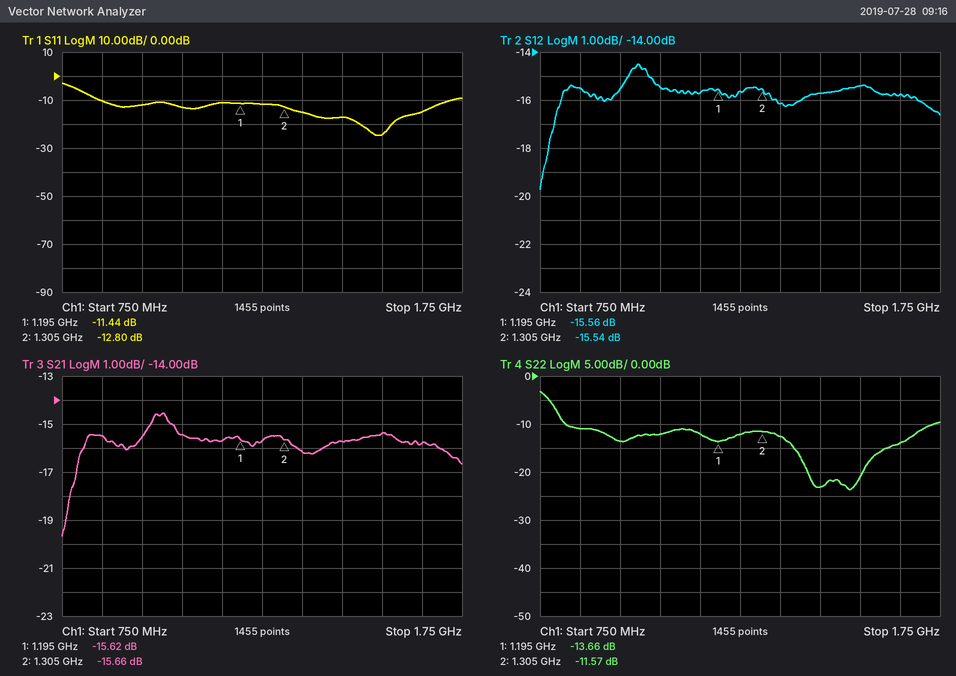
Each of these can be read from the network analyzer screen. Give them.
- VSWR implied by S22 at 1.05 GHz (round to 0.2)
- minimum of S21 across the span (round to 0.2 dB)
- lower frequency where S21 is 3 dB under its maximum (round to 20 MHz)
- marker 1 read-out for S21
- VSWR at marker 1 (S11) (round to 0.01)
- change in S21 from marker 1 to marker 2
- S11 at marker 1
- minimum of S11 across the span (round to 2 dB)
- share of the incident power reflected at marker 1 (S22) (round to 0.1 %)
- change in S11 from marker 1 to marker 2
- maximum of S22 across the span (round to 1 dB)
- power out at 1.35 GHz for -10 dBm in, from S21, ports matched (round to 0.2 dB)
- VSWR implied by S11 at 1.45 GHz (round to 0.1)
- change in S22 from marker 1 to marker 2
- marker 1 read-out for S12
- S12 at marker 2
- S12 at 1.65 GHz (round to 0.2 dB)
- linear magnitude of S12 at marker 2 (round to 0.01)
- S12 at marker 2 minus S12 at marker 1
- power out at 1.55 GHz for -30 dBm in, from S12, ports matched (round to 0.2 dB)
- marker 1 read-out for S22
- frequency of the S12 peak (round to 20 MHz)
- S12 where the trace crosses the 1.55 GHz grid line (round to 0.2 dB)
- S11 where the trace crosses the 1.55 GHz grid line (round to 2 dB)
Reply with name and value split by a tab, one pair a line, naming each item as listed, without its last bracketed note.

VSWR implied by S22 at 1.05 GHz	1.6
minimum of S21 across the span	-19.6 dB
lower frequency where S21 is 3 dB under its maximum	780 MHz
marker 1 read-out for S21	-15.62 dB
VSWR at marker 1 (S11)	1.73
change in S21 from marker 1 to marker 2	-0.04 dB
S11 at marker 1	-11.44 dB
minimum of S11 across the span	-24 dB
share of the incident power reflected at marker 1 (S22)	4.3 %
change in S11 from marker 1 to marker 2	-1.36 dB
maximum of S22 across the span	-3 dB
power out at 1.35 GHz for -10 dBm in, from S21, ports matched	-26.2 dBm
VSWR implied by S11 at 1.45 GHz	1.3
change in S22 from marker 1 to marker 2	2.09 dB
marker 1 read-out for S12	-15.56 dB
S12 at marker 2	-15.54 dB
S12 at 1.65 GHz	-15.8 dB
linear magnitude of S12 at marker 2	0.17
S12 at marker 2 minus S12 at marker 1	0.02 dB
power out at 1.55 GHz for -30 dBm in, from S12, ports matched	-45.4 dBm
marker 1 read-out for S22	-13.66 dB
frequency of the S12 peak	1.00 GHz
S12 where the trace crosses the 1.55 GHz grid line	-15.4 dB
S11 where the trace crosses the 1.55 GHz grid line	-24 dB
